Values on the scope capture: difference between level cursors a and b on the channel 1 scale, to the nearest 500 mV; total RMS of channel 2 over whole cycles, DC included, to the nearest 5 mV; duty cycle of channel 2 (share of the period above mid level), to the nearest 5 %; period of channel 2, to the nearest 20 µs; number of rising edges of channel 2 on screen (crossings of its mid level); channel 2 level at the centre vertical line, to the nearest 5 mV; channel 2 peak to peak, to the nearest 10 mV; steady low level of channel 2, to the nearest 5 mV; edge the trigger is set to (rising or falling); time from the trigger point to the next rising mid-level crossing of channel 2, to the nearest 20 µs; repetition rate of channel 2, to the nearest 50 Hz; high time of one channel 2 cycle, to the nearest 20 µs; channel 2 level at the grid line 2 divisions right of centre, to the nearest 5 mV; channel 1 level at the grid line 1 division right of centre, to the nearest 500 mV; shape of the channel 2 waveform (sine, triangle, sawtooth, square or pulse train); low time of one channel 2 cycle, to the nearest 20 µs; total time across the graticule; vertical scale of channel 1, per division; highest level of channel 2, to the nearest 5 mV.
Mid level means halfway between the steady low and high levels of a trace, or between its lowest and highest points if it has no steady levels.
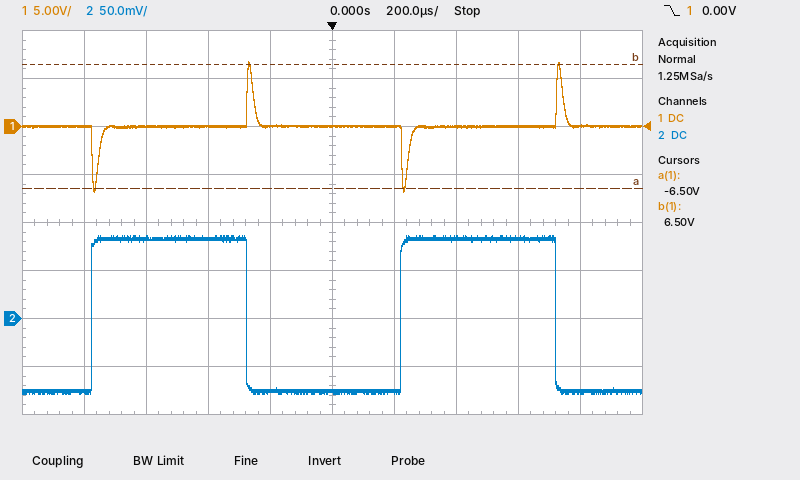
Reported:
13.0 V
80 mV
50 %
1.00 ms
2
-75 mV
160 mV
-75 mV
falling
220 µs
1.00 kHz
500 µs
85 mV
0.0 V
square
500 µs
2 ms
5 V
85 mV
